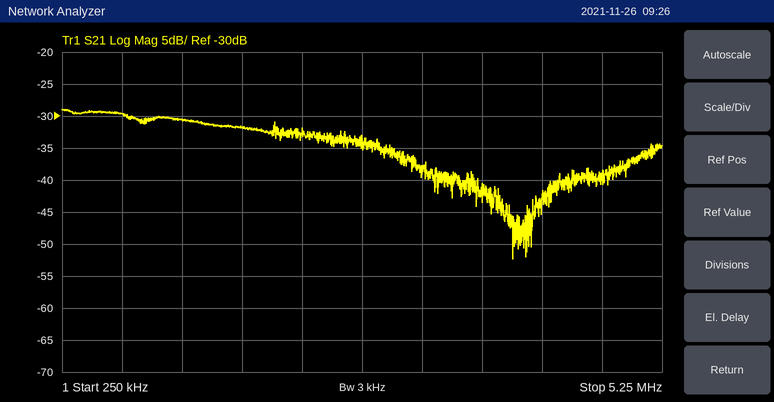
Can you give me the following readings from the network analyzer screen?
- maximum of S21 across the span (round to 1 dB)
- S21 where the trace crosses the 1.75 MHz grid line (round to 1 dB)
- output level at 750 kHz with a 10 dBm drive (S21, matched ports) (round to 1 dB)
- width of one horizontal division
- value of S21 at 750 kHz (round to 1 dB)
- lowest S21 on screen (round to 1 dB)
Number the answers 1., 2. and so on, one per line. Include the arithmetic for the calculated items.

1. -29 dB
2. -32 dB
3. 10 dBm + (-30 dB) = -20 dBm
4. 500 kHz
5. -30 dB
6. -52 dB
